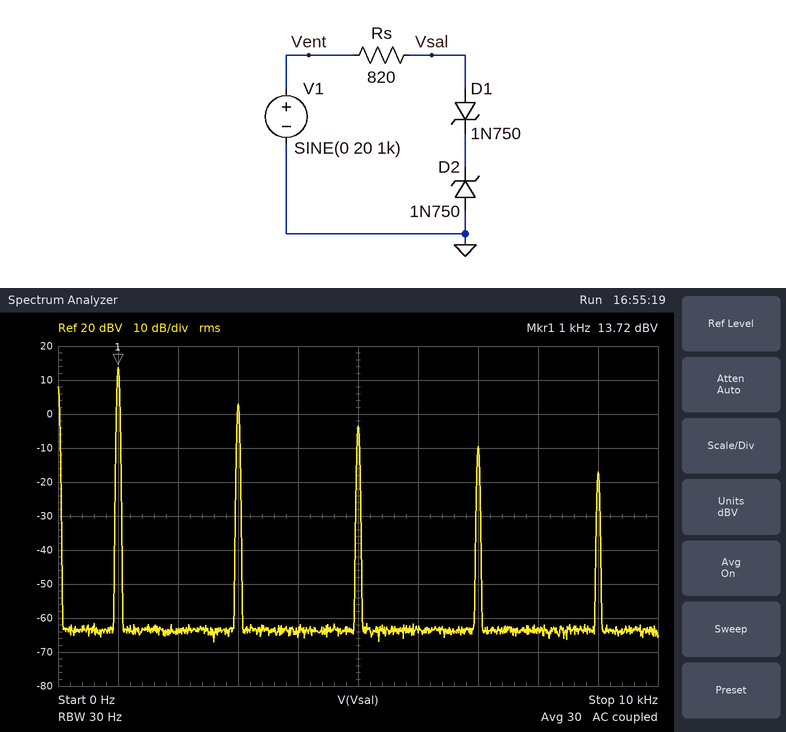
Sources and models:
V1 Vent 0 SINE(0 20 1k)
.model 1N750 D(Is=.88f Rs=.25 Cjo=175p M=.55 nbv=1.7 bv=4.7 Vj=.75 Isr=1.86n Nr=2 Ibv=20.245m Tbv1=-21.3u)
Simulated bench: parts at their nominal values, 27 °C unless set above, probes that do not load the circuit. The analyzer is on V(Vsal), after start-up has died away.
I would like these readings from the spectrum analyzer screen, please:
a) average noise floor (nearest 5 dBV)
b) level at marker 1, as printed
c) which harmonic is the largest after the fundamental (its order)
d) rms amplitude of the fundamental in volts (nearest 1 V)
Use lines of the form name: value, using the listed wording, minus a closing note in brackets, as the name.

average noise floor: -65 dBV
level at marker 1, as printed: 13.72 dBV
which harmonic is the largest after the fundamental: 3
rms amplitude of the fundamental in volts: 5 V
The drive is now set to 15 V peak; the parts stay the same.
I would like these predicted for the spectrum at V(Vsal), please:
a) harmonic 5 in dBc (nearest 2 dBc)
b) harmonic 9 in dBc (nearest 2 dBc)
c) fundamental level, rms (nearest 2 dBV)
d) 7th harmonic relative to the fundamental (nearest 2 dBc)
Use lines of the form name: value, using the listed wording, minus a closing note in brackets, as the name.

harmonic 5 in dBc: -20 dBc
harmonic 9 in dBc: -56 dBc
fundamental level, rms: 14 dBV
7th harmonic relative to the fundamental: -30 dBc
